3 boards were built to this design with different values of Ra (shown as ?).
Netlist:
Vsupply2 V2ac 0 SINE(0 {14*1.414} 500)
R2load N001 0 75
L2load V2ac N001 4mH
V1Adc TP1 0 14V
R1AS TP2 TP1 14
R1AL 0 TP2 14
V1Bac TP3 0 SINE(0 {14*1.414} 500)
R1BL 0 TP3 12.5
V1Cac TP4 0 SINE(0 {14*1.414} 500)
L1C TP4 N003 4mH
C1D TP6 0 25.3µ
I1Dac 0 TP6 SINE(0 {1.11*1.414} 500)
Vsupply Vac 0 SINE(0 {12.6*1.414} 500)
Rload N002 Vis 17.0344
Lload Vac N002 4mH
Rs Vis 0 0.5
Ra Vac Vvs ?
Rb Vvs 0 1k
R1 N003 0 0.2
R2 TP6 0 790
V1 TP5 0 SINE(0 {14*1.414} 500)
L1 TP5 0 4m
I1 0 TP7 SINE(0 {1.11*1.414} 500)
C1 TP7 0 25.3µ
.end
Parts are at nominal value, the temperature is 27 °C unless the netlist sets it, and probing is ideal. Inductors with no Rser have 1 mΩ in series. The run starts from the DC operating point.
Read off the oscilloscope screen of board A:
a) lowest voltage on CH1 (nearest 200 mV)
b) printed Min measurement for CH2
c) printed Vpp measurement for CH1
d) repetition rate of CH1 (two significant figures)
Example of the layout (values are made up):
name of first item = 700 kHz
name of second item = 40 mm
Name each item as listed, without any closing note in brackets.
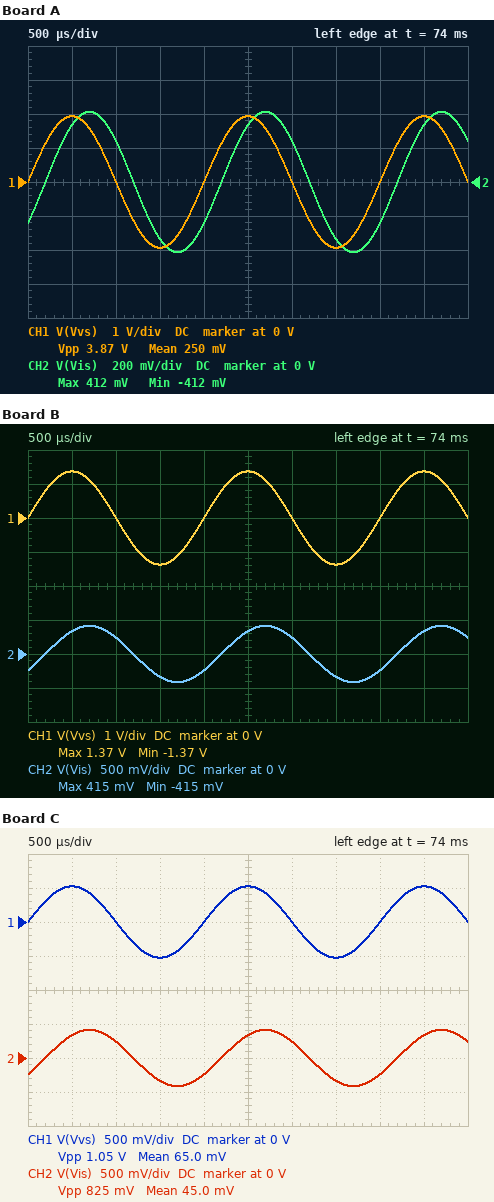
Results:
lowest voltage on CH1 = -2.0 V
printed Min measurement for CH2 = -412 mV
printed Vpp measurement for CH1 = 3.87 V
repetition rate of CH1 = 500 Hz
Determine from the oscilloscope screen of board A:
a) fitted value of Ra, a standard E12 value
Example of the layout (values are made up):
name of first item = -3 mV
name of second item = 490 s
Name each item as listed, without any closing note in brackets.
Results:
fitted value of Ra, a standard E12 value = 8.2 kΩ
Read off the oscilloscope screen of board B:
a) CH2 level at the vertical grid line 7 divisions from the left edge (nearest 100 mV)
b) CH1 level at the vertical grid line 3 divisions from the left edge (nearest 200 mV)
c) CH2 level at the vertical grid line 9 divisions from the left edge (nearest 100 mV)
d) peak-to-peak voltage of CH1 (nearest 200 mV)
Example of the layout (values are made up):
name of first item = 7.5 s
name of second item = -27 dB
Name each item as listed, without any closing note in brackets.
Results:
CH2 level at the vertical grid line 7 divisions from the left edge = -300 mV
CH1 level at the vertical grid line 3 divisions from the left edge = -1.4 V
CH2 level at the vertical grid line 9 divisions from the left edge = 300 mV
peak-to-peak voltage of CH1 = 2.8 V
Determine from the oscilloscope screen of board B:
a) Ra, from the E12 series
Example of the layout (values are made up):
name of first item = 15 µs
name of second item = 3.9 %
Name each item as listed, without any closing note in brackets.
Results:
Ra, from the E12 series = 12 kΩ
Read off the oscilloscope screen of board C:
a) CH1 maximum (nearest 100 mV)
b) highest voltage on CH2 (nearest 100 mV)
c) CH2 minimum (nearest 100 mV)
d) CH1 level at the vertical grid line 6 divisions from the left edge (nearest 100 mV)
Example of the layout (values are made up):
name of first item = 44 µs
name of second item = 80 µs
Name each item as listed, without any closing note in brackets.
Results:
CH1 maximum = 500 mV
highest voltage on CH2 = 400 mV
CH2 minimum = -400 mV
CH1 level at the vertical grid line 6 divisions from the left edge = 0 V
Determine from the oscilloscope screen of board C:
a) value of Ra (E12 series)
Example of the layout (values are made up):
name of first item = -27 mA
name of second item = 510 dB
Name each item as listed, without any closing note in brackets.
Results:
value of Ra = 33 kΩ
